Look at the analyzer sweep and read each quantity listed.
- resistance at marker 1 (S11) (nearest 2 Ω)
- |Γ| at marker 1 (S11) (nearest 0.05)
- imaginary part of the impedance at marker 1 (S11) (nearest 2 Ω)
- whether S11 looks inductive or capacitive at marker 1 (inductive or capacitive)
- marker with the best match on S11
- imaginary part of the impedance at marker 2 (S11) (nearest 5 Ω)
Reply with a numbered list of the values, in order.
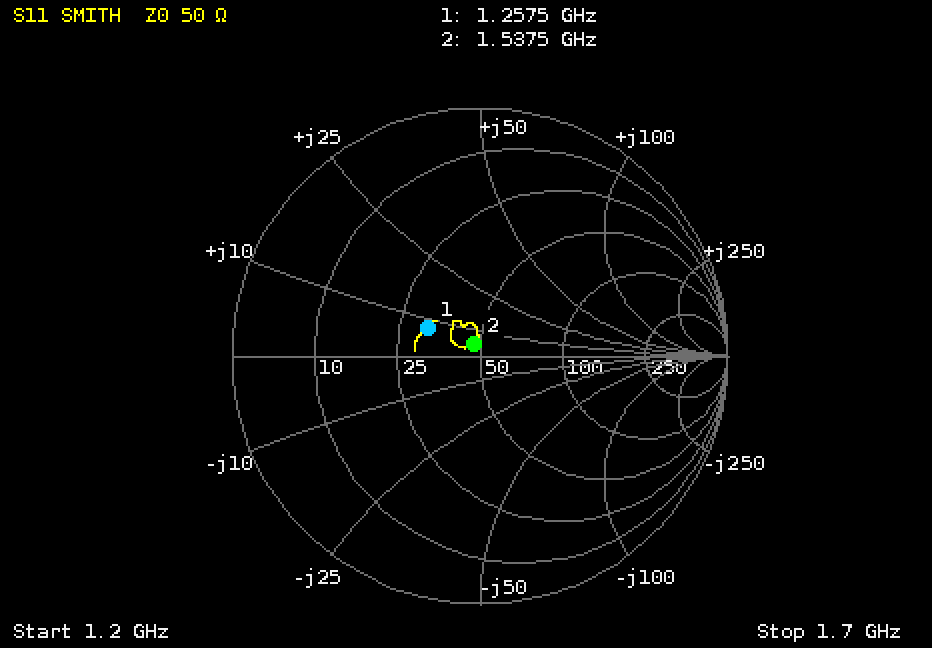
1. 32 Ω
2. 0.25
3. +8 Ω
4. inductive
5. marker 2
6. +5 Ω
